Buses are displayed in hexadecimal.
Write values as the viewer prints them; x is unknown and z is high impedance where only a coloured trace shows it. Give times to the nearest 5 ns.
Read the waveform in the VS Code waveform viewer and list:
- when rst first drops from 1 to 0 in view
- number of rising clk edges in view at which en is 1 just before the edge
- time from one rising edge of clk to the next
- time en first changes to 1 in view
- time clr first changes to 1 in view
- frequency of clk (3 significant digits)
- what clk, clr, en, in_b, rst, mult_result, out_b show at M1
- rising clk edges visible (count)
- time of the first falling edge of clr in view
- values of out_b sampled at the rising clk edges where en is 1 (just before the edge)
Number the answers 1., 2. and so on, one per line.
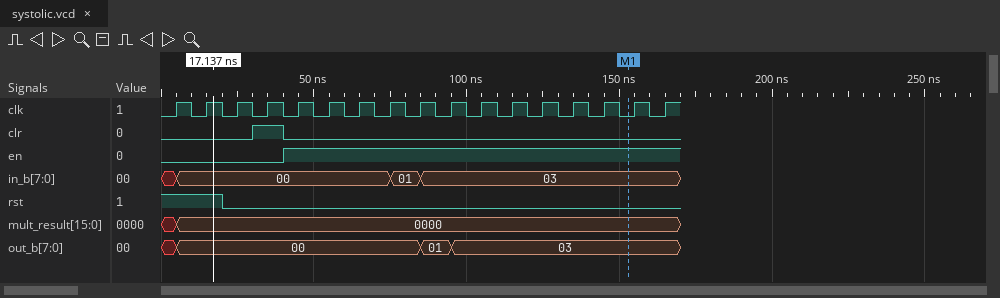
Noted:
1. 20 ns
2. 13
3. 10 ns
4. 40 ns
5. 30 ns
6. 100 MHz
7. clk=0, clr=0, en=1, in_b=03, rst=0, mult_result=0000, out_b=03
8. 17
9. 40 ns
10. 00, 00, 00, 00, 00, 01, 03, 03, 03, 03, 03, 03, 03
